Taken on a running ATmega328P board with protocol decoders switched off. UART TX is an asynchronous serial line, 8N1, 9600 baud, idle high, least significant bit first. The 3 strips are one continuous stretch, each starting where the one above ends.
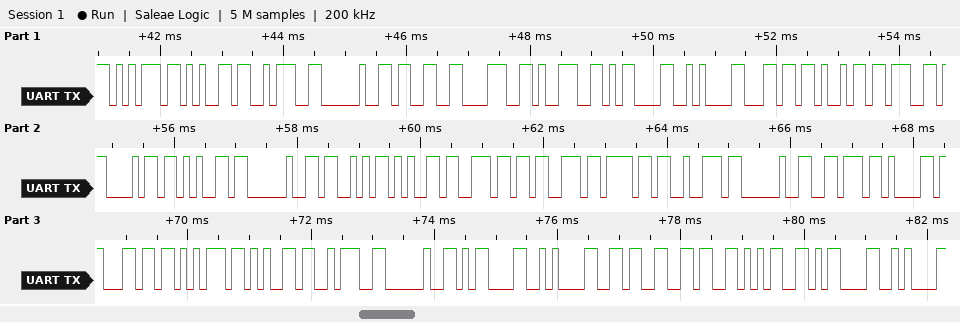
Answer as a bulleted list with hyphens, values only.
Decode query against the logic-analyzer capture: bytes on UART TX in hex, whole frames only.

- 75 65 3A 20 33 38 39 0D 0A 6C 69 67 68 65 20 53 65 6E 73 6F 72 20 76 61 6C 75 65 3A 20 0D 0A 36 36 35 0D 0A
